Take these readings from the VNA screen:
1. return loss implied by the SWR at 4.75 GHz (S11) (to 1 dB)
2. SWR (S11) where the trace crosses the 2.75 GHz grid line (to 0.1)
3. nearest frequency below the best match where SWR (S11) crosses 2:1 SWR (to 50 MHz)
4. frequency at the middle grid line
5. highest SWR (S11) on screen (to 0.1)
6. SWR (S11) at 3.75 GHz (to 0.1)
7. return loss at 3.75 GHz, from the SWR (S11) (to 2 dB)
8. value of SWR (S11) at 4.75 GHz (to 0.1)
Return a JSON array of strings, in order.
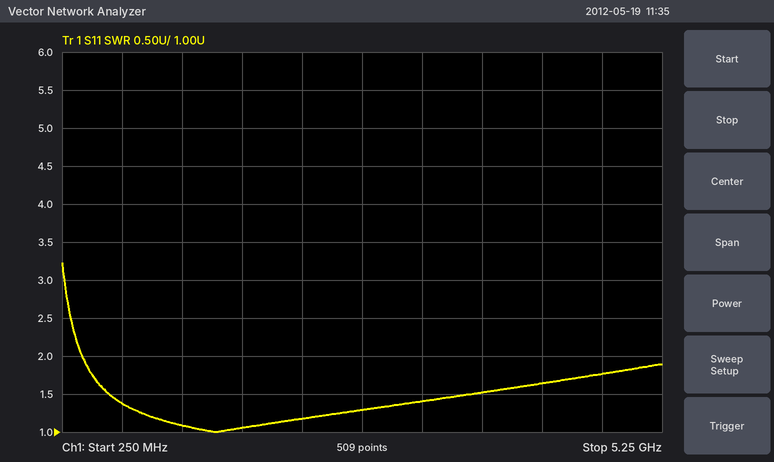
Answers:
["11 dB", "1.3", "400 MHz", "2.75 GHz", "3.2", "1.5", "14 dB", "1.8"]
